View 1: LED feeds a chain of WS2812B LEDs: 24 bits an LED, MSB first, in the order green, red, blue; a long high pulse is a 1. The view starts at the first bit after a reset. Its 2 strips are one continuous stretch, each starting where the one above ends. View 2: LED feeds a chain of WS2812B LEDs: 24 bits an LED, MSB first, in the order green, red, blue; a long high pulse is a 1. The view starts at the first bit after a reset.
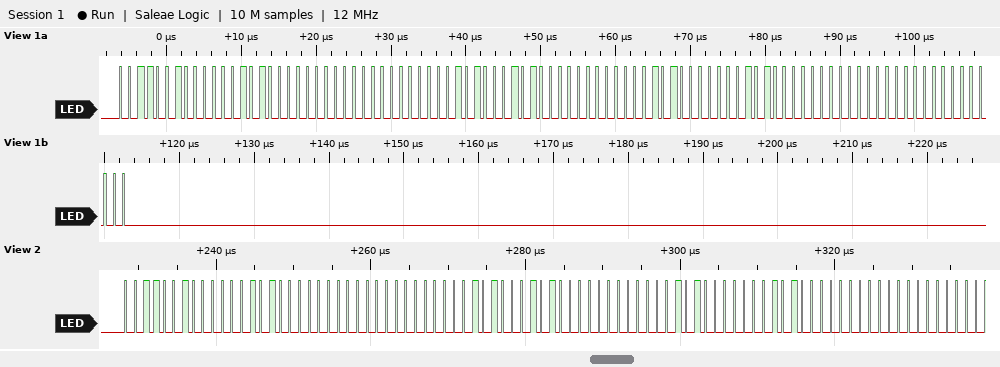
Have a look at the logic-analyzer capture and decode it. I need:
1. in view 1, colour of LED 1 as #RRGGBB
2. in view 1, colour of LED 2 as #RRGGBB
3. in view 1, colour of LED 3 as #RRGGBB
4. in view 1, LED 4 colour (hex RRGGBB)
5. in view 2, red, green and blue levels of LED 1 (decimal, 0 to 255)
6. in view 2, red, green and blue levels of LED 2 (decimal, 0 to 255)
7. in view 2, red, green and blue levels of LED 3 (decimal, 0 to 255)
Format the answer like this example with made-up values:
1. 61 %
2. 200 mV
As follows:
1. #053200
2. #0A0028
3. #500014
4. #000000
5. 5, 50, 0
6. 10, 0, 40
7. 80, 0, 20
